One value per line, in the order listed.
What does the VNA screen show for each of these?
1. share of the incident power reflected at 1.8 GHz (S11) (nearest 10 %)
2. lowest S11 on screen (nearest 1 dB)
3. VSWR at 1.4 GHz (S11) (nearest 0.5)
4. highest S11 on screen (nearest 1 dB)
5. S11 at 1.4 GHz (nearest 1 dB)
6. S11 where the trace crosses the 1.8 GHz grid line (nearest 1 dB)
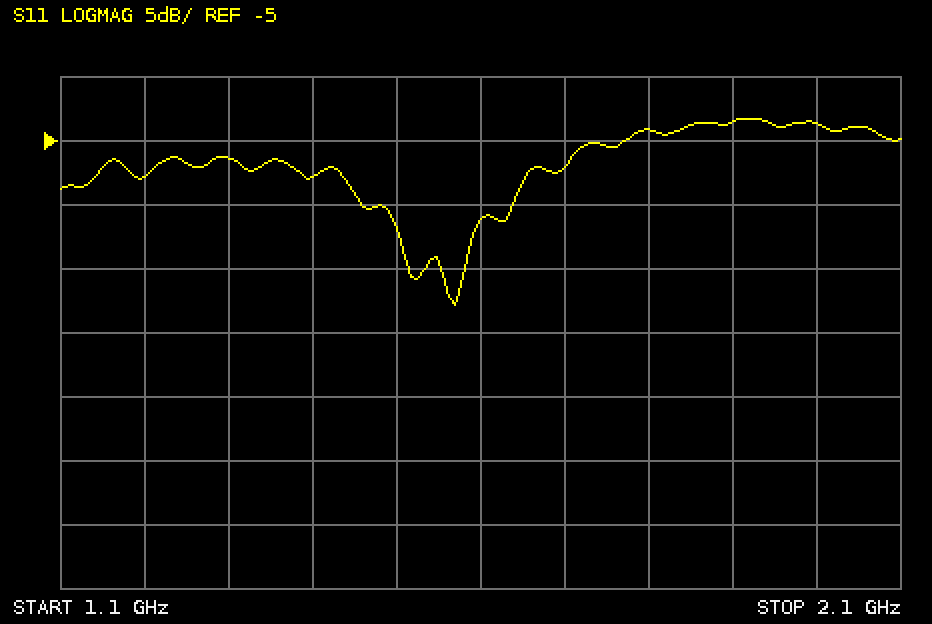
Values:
40 %
-18 dB
2.5
-3 dB
-8 dB
-4 dB
